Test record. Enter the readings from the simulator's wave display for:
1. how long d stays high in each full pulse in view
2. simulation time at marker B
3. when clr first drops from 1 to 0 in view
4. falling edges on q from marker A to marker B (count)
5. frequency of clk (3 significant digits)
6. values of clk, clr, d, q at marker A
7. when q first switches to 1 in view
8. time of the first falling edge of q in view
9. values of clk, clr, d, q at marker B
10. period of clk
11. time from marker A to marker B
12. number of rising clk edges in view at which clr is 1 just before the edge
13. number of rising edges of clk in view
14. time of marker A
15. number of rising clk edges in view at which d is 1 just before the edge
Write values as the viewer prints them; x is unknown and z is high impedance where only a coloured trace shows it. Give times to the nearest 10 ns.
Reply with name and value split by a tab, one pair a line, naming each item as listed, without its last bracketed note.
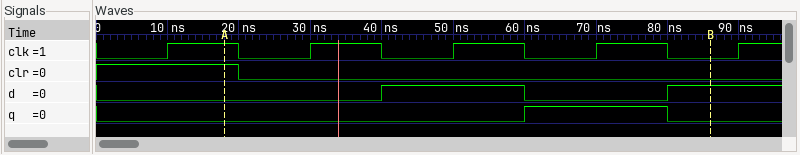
how long d stays high in each full pulse in view	20 ns
simulation time at marker B	90 ns
when clr first drops from 1 to 0 in view	20 ns
falling edges on q from marker A to marker B	1
frequency of clk	50.0 MHz
values of clk, clr, d, q at marker A	clk=1, clr=1, d=0, q=0
when q first switches to 1 in view	60 ns
time of the first falling edge of q in view	80 ns
values of clk, clr, d, q at marker B	clk=0, clr=0, d=1, q=0
period of clk	20 ns
time from marker A to marker B	70 ns
number of rising clk edges in view at which clr is 1 just before the edge	1
number of rising edges of clk in view	5
time of marker A	20 ns
number of rising clk edges in view at which d is 1 just before the edge	2
